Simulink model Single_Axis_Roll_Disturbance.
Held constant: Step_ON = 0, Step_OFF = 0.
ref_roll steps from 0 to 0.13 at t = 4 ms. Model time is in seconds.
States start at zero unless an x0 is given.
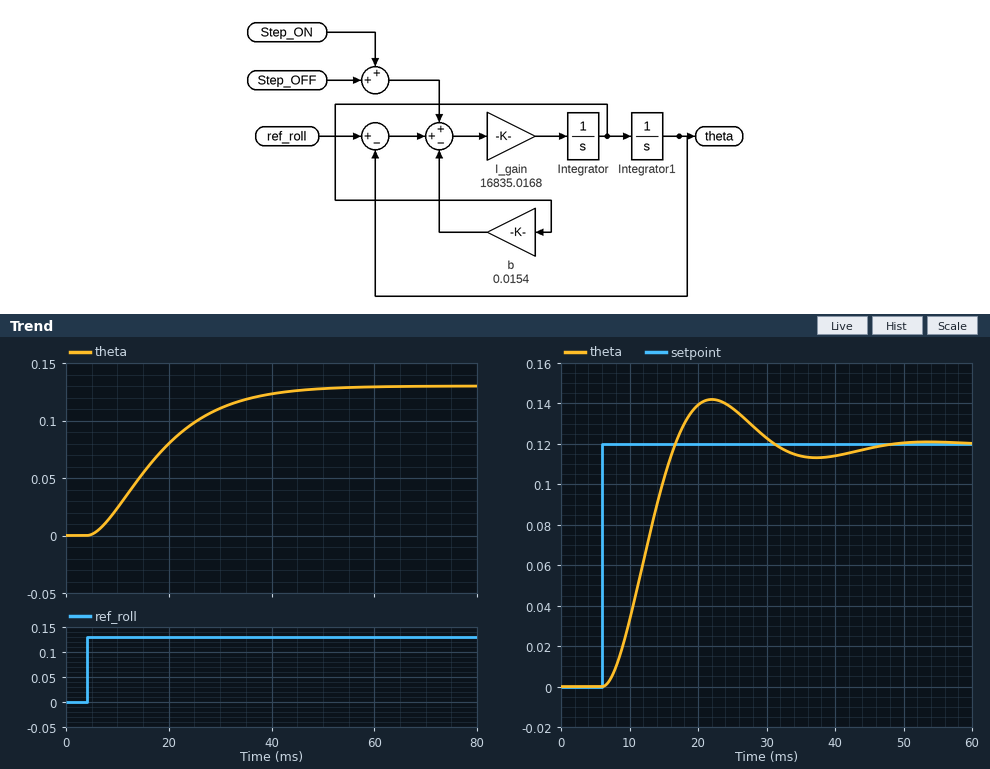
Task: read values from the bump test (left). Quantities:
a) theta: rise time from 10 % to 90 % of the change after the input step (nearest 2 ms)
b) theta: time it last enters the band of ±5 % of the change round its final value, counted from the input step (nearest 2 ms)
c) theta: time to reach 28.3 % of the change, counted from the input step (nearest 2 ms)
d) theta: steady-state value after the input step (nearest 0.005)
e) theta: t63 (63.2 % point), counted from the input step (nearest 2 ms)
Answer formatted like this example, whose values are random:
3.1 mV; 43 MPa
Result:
26 ms; 36 ms; 8 ms; 0.130; 16 ms
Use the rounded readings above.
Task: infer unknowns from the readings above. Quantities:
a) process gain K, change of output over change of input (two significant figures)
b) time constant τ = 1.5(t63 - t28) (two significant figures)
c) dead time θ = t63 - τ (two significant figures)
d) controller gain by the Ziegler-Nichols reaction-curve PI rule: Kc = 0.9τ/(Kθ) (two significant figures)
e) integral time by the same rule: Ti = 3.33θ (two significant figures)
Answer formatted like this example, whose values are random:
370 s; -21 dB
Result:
1.0; 12 ms; 4.0 ms; 2.7; 13 ms
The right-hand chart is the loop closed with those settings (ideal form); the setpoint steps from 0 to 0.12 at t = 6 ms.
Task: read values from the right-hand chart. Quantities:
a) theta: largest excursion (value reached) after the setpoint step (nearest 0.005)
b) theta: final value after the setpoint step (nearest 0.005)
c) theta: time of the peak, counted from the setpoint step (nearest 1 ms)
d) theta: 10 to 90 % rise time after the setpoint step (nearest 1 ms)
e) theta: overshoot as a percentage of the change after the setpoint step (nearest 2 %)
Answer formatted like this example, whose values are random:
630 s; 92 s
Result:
0.140; 0.120; 16 ms; 7 ms; 18 %
